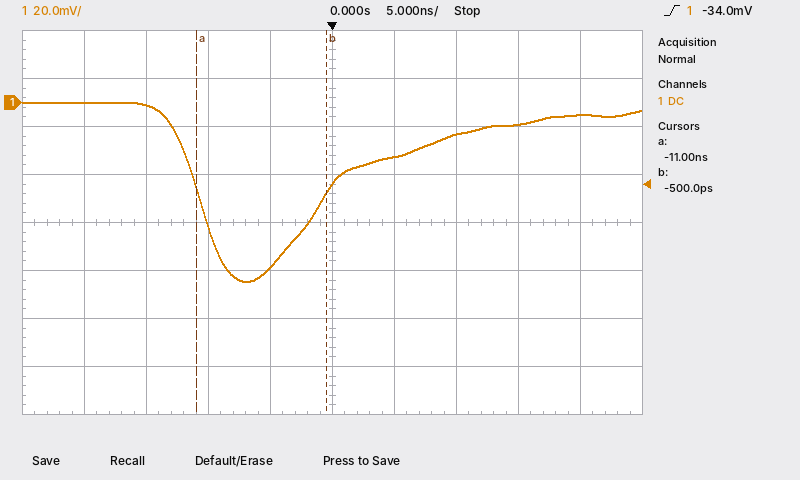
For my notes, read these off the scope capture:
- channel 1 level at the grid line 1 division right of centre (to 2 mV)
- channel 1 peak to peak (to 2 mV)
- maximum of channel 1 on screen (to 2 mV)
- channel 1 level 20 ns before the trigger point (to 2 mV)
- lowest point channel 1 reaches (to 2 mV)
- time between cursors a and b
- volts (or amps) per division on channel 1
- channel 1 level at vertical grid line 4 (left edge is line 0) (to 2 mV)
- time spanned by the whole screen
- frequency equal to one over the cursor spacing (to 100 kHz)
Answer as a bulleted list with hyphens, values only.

- -22 mV
- 74 mV
- 0 mV
- 0 mV
- -74 mV
- 10.5 ns
- 20 mV
- -68 mV
- 50 ns
- 95.2 MHz
